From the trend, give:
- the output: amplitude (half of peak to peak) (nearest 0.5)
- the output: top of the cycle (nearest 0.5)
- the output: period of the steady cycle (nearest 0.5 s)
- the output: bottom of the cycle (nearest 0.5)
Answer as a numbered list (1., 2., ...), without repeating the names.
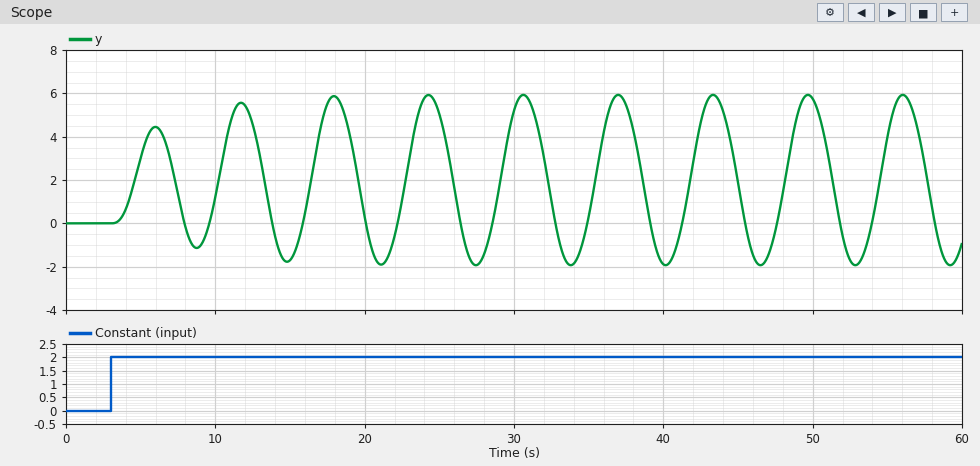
1. 4.0
2. 6.0
3. 6.5 s
4. -2.0
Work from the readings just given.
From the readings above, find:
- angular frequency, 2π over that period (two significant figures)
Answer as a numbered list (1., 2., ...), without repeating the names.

1. 0.97 rad/s
